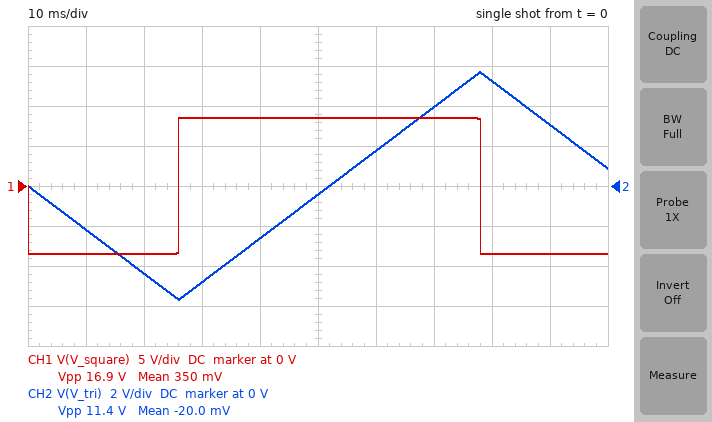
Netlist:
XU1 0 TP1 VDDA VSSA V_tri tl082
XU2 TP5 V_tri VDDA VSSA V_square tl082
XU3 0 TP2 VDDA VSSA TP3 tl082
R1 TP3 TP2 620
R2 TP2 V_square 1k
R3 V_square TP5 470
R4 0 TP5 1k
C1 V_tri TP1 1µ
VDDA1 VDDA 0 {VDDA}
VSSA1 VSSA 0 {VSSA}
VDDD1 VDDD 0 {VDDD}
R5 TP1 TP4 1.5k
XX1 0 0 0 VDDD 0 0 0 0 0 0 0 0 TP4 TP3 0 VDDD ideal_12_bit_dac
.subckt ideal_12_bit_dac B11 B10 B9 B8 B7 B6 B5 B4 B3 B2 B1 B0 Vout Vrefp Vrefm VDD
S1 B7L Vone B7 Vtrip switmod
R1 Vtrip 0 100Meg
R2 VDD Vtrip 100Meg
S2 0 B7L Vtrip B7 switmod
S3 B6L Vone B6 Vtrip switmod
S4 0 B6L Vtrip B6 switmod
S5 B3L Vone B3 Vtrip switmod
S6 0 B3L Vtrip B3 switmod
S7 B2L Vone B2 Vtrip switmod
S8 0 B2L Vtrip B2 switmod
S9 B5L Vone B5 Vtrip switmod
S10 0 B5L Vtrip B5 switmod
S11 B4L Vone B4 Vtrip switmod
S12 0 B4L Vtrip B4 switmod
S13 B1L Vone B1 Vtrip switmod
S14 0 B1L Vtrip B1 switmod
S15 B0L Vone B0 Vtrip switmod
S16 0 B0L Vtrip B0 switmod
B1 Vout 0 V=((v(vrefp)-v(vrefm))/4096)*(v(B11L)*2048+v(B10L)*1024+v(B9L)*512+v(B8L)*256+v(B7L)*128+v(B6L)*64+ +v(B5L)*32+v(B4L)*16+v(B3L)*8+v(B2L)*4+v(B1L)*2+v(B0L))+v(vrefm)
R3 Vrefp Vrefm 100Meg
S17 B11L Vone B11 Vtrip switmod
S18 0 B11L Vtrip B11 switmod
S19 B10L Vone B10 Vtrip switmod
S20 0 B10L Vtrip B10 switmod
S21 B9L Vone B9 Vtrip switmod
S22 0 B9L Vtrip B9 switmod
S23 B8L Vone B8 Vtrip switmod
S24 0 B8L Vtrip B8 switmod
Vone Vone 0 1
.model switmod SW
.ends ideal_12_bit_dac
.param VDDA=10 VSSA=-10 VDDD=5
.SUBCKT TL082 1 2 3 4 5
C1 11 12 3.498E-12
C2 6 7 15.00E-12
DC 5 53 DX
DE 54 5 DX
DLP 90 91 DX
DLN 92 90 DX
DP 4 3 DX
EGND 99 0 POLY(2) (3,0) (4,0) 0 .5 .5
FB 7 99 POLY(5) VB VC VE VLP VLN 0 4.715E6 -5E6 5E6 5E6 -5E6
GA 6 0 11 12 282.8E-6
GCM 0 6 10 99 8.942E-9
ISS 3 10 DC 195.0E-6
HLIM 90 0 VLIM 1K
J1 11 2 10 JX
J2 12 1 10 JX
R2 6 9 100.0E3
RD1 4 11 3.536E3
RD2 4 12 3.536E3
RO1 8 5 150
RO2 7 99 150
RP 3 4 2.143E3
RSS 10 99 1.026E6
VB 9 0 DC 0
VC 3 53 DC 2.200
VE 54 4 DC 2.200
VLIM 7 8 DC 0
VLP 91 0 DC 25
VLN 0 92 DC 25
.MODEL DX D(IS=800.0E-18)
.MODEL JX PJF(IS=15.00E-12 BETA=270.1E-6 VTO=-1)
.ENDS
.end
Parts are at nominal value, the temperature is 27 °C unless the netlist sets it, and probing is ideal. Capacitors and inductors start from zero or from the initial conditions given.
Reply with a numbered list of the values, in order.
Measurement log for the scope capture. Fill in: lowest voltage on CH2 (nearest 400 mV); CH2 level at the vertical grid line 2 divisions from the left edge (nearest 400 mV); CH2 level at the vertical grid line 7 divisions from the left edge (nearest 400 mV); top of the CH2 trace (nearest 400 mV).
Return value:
1. -5.6 V
2. -4.4 V
3. 4.0 V
4. 5.6 V
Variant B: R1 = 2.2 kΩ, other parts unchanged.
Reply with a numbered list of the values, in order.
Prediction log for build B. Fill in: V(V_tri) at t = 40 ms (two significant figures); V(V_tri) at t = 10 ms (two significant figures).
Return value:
1. 2.7 V
2. -3.5 V
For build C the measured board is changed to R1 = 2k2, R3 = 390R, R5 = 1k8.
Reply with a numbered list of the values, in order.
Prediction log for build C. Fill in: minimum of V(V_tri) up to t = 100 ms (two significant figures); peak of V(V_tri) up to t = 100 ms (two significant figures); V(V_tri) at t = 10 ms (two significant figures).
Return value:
1. -6.0 V
2. 6.0 V
3. -2.9 V
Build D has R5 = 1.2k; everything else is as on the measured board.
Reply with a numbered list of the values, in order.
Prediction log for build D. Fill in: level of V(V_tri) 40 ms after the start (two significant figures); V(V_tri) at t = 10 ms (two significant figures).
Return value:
1. -430 mV
2. -2.7 V
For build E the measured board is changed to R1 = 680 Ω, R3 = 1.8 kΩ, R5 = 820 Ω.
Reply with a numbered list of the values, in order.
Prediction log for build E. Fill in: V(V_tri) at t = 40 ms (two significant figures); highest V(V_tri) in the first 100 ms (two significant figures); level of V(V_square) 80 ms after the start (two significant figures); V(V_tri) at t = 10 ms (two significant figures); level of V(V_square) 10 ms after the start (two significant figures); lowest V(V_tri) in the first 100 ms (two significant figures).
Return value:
1. -340 mV
2. 3.0 V
3. -8.5 V
4. -1.6 V
5. 8.5 V
6. -3.0 V
